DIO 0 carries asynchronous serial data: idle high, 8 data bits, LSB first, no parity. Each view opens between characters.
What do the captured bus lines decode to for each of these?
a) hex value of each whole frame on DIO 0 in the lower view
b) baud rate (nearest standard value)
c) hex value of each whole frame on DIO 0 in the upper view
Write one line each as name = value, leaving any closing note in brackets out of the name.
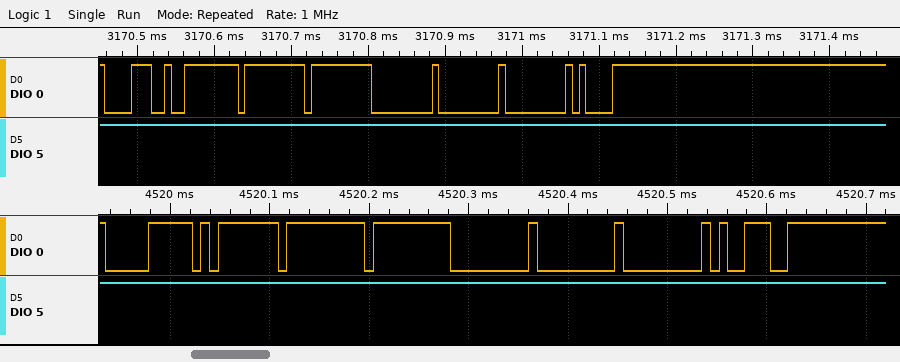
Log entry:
hex value of each whole frame on DIO 0 in the lower view = F0, FD, FF, FF, 00, 00, 00, 39
baud rate = 115200 baud
hex value of each whole frame on DIO 0 in the upper view = 38, FE, FF, FF, 00, 00, 00, E1
